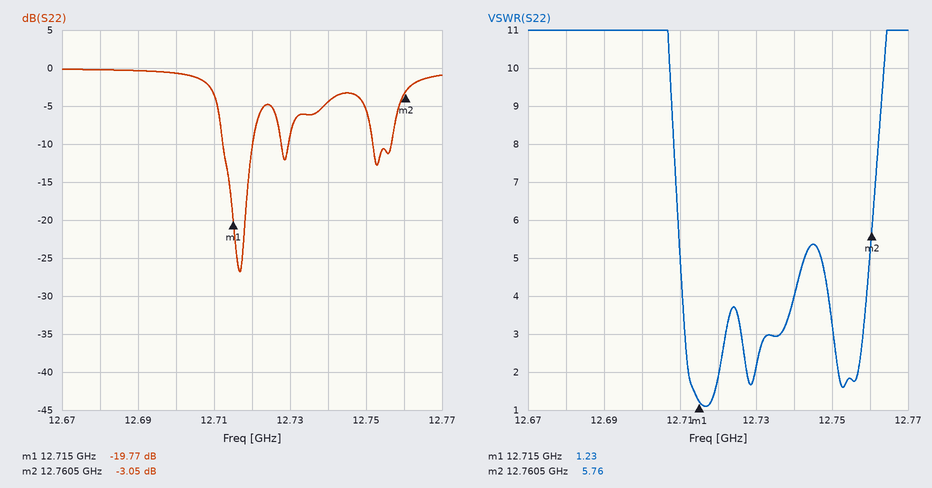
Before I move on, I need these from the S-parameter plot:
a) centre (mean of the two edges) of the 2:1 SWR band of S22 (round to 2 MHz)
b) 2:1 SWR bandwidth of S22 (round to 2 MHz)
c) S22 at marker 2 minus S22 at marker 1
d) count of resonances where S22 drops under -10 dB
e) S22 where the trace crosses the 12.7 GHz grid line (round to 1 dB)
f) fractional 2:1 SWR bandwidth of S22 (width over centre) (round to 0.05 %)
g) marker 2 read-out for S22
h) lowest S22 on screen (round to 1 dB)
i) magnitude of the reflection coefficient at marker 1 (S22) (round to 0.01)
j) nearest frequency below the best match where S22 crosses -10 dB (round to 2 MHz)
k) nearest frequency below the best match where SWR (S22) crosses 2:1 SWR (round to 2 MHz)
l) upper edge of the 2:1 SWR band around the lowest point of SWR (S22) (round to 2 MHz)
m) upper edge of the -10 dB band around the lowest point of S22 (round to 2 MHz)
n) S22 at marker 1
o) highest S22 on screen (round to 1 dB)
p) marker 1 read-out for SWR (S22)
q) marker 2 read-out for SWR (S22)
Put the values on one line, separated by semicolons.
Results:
12.716 GHz; 8 MHz; 16.72 dB; 3; -1 dB; 0.05 %; -3.05 dB; -27 dB; 0.10; 12.712 GHz; 12.712 GHz; 12.720 GHz; 12.720 GHz; -19.77 dB; 0 dB; 1.23; 5.76
